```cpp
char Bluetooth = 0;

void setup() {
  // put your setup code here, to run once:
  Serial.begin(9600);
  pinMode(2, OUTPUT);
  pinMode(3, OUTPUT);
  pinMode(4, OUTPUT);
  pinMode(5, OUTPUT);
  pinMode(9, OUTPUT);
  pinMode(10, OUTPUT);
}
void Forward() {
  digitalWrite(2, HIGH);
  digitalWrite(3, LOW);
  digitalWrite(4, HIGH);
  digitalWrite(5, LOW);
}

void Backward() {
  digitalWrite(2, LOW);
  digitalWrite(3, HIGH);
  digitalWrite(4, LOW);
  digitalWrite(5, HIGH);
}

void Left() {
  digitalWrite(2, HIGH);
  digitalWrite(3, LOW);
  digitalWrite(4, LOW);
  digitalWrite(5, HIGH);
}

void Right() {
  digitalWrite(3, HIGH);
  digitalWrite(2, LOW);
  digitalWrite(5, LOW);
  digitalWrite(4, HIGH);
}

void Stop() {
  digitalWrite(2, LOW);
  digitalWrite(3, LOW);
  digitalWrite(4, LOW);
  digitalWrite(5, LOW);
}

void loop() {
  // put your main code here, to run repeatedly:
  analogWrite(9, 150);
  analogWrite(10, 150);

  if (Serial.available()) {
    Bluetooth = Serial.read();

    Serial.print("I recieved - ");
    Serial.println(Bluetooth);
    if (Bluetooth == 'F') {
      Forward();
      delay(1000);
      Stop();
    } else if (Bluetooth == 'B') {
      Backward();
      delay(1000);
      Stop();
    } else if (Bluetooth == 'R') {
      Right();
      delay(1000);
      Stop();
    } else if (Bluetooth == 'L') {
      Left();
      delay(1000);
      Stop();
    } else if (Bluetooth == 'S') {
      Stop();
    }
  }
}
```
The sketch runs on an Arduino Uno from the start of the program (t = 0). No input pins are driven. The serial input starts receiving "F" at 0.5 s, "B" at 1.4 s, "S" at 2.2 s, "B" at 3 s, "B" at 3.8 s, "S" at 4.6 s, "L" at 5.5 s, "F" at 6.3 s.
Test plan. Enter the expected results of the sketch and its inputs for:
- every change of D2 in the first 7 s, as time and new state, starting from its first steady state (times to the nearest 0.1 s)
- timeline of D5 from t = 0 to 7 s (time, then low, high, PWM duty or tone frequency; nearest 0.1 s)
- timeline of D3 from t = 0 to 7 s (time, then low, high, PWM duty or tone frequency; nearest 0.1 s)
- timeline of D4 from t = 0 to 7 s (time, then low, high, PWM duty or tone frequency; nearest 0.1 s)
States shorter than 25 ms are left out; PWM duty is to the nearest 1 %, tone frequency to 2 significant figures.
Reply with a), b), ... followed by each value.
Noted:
a) 0 s low; 0.5 s high; 1.5 s low; 5.5 s high
b) 0 s low; 1.5 s high; 2.5 s low; 3 s high; 5 s low; 5.5 s high; 6.5 s low
c) 0 s low; 1.5 s high; 2.5 s low; 3 s high; 5 s low
d) 0 s low; 0.5 s high; 1.5 s low; 6.5 s high
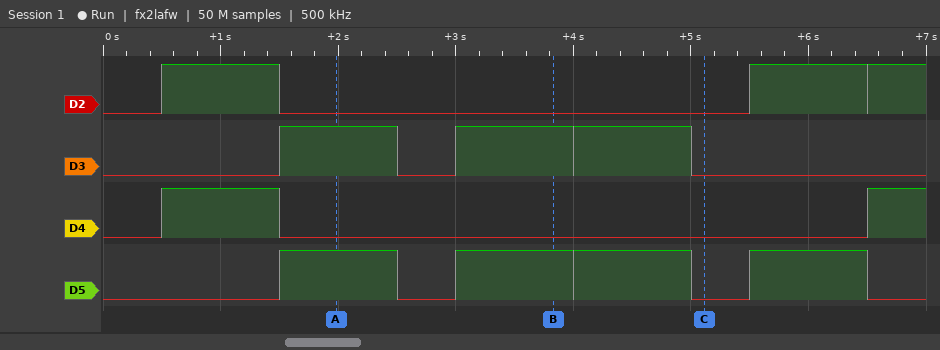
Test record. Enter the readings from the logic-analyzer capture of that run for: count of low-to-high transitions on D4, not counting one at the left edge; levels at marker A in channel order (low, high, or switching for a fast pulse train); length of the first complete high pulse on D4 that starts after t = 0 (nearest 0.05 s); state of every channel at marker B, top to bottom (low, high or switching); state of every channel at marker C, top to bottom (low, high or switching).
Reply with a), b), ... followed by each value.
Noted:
a) 2
b) D2 low, D3 high, D4 low, D5 high
c) 1.00 s
d) D2 low, D3 high, D4 low, D5 high
e) D2 low, D3 low, D4 low, D5 low
